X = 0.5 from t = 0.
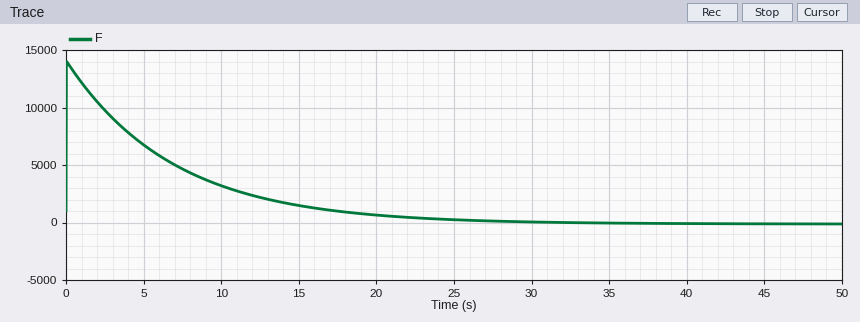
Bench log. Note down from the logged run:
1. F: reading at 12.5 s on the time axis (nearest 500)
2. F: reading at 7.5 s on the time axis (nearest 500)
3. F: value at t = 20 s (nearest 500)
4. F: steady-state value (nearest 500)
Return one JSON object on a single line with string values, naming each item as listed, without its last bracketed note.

{"F: reading at 12.5 s on the time axis": "2000", "F: reading at 7.5 s on the time axis": "4500", "F: value at t = 20 s": "500", "F: steady-state value": "0"}
